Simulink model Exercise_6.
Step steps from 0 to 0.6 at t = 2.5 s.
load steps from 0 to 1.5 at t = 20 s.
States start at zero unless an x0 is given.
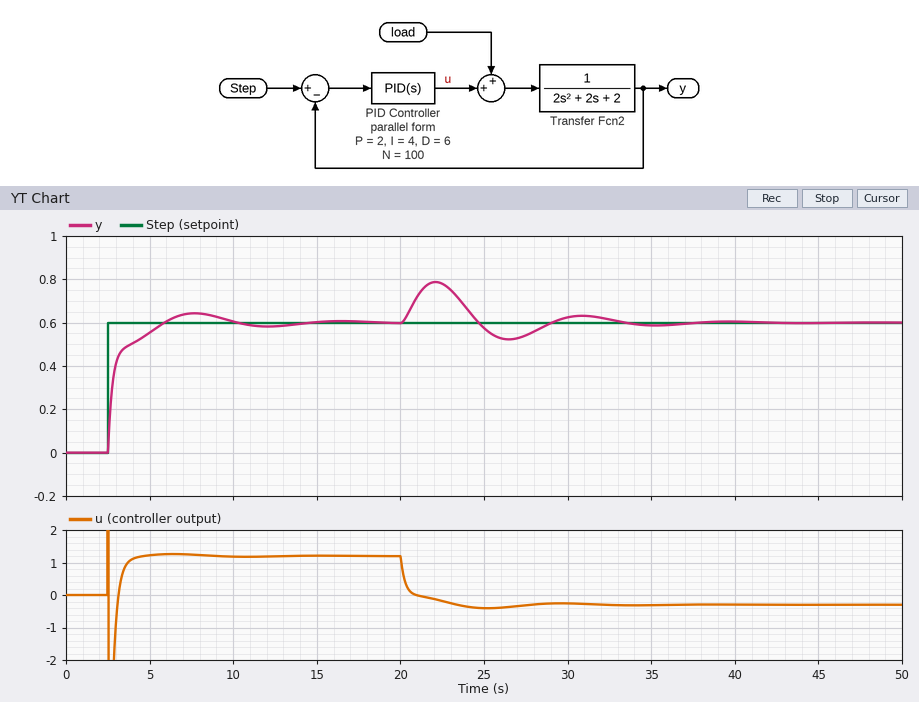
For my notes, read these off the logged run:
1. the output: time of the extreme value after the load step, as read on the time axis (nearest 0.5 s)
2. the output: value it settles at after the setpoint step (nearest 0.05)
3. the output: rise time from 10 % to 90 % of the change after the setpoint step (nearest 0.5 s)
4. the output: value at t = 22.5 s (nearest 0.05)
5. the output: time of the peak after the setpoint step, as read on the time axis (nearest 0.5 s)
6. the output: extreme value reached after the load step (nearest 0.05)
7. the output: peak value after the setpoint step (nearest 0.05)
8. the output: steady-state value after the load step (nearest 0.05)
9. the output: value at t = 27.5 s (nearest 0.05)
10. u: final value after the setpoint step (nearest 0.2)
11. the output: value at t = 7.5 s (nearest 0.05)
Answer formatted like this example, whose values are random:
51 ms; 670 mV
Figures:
22.0 s; 0.60; 2.0 s; 0.80; 7.5 s; 0.80; 0.65; 0.60; 0.55; 1.2; 0.65
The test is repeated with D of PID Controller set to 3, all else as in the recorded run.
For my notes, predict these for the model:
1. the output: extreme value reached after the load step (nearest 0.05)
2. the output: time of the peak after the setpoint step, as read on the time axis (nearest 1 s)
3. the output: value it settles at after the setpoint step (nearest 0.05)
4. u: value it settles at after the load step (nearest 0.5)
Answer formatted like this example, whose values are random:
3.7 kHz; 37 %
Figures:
0.85; 6 s; 0.60; -0.5
